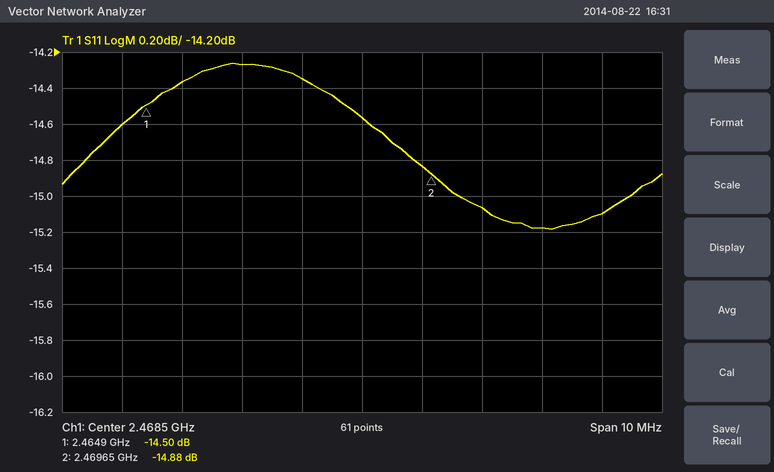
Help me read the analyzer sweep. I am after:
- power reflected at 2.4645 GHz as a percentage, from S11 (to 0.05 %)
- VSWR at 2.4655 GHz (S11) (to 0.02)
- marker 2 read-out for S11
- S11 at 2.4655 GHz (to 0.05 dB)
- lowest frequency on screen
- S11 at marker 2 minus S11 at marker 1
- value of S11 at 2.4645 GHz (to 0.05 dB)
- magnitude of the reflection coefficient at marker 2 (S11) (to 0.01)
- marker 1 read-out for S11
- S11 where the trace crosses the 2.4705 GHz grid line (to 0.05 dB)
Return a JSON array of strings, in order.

["3.45 %", "1.48", "-14.88 dB", "-14.35 dB", "2.4635 GHz", "-0.38 dB", "-14.60 dB", "0.18", "-14.50 dB", "-15.05 dB"]
